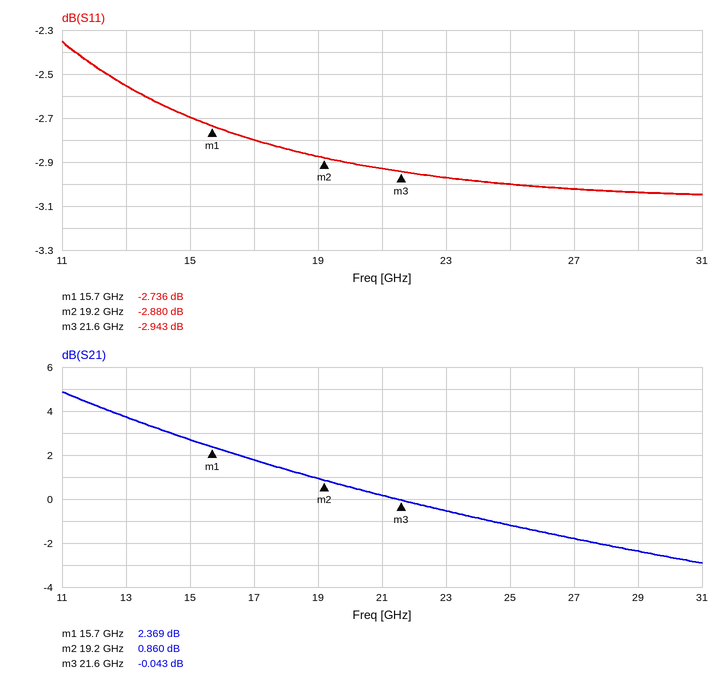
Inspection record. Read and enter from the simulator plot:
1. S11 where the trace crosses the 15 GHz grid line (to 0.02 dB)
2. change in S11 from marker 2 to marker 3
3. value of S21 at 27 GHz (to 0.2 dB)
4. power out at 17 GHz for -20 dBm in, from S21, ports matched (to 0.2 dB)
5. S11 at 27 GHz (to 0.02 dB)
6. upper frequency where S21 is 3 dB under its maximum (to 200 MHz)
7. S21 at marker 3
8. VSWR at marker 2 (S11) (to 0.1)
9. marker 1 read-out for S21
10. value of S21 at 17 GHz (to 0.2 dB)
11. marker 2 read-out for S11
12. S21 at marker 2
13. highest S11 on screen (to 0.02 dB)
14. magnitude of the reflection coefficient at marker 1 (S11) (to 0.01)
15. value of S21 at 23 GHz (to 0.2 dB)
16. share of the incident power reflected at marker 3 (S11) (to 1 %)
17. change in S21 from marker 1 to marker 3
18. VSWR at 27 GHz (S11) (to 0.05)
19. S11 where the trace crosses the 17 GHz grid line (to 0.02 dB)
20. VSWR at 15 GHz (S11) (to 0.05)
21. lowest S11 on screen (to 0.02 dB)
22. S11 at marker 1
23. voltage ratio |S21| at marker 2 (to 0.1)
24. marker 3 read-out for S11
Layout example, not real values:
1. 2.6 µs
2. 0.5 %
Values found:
1. -2.70 dB
2. -0.063 dB
3. -1.8 dB
4. -18.2 dBm
5. -3.02 dB
6. 16.8 GHz
7. -0.043 dB
8. 6.1
9. 2.369 dB
10. 1.8 dB
11. -2.880 dB
12. 0.860 dB
13. -2.36 dB
14. 0.73
15. -0.6 dB
16. 51 %
17. -2.412 dB
18. 5.80
19. -2.80 dB
20. 6.50
21. -3.04 dB
22. -2.736 dB
23. 1.1
24. -2.943 dB
